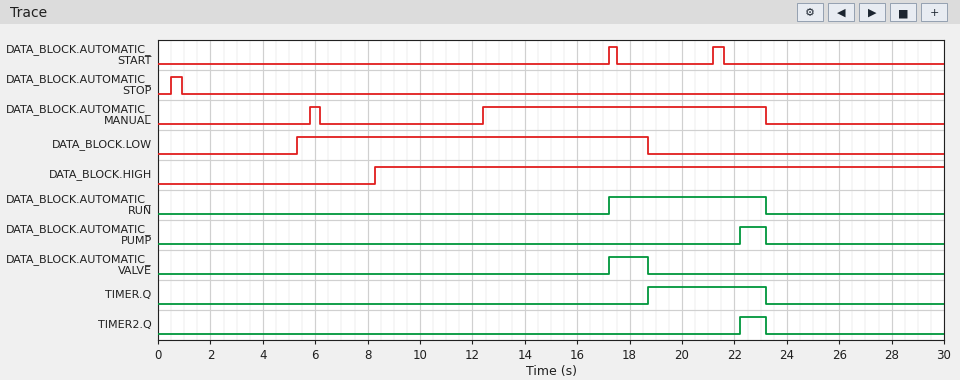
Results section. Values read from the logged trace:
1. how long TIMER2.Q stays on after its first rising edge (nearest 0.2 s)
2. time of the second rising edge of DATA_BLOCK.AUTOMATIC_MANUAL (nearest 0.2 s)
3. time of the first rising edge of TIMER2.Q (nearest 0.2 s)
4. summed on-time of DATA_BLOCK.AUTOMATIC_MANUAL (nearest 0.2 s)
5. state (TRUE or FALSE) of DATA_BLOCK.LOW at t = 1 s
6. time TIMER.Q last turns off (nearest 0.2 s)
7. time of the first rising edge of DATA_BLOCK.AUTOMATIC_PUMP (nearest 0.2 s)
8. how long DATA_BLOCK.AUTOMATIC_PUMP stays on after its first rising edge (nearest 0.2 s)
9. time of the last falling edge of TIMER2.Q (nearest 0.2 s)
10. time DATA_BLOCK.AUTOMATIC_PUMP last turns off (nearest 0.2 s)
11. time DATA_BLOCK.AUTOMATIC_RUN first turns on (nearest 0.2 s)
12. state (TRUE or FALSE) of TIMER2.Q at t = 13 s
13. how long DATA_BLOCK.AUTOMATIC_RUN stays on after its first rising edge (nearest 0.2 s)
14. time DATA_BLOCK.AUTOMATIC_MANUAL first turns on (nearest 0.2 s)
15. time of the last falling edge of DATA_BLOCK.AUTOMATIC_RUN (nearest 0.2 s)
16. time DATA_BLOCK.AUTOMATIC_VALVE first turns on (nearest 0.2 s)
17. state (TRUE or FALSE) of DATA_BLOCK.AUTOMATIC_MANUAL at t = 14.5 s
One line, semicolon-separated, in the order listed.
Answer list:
1.0 s; 12.4 s; 22.2 s; 11.2 s; FALSE; 23.2 s; 22.2 s; 1.0 s; 23.2 s; 23.2 s; 17.2 s; FALSE; 6.0 s; 5.8 s; 23.2 s; 17.2 s; TRUE
